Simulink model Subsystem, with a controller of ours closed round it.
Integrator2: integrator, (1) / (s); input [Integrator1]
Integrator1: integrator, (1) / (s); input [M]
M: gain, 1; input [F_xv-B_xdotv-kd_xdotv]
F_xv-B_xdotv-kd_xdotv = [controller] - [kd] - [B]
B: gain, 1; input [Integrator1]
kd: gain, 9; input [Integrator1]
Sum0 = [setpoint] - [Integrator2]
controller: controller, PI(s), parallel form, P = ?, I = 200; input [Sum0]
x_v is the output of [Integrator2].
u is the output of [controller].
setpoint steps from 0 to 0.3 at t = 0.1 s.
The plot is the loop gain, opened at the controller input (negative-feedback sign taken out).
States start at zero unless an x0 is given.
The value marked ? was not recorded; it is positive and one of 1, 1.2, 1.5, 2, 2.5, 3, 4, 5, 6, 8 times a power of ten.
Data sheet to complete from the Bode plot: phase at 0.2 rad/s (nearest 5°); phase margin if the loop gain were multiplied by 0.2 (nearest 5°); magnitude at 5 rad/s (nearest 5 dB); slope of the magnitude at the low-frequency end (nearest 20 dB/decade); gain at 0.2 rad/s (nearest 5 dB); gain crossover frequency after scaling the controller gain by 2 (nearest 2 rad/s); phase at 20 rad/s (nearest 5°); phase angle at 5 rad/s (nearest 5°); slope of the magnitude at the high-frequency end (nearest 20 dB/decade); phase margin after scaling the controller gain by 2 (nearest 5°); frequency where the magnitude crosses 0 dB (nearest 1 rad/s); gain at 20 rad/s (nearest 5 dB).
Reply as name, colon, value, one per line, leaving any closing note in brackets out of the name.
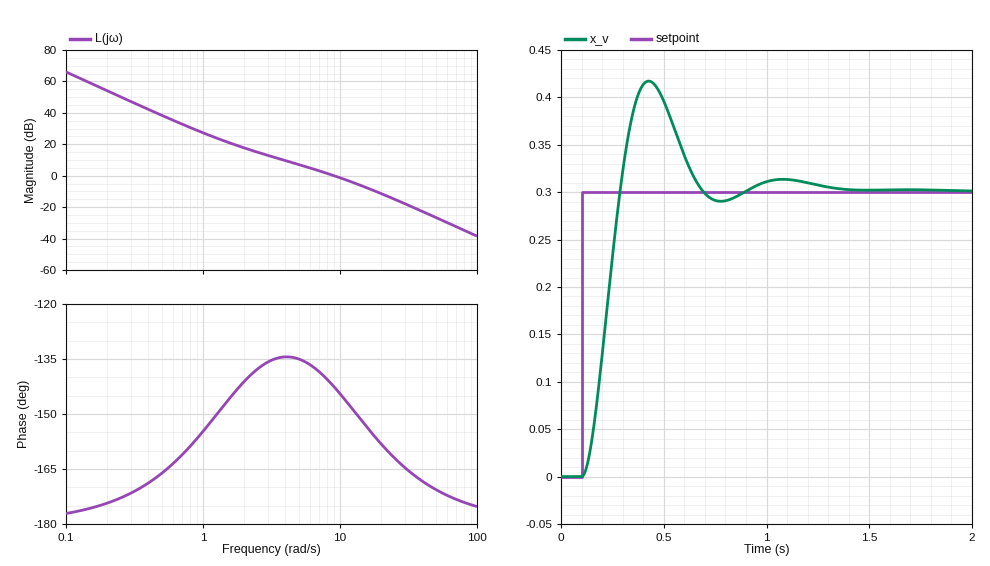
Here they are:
phase at 0.2 rad/s: -175°
phase margin if the loop gain were multiplied by 0.2: 45°
magnitude at 5 rad/s: 5 dB
slope of the magnitude at the low-frequency end: -40 dB/decade
gain at 0.2 rad/s: 55 dB
gain crossover frequency after scaling the controller gain by 2: 14 rad/s
phase at 20 rad/s: -160°
phase angle at 5 rad/s: -135°
slope of the magnitude at the high-frequency end: -40 dB/decade
phase margin after scaling the controller gain by 2: 30°
frequency where the magnitude crosses 0 dB: 9 rad/s
gain at 20 rad/s: -10 dB
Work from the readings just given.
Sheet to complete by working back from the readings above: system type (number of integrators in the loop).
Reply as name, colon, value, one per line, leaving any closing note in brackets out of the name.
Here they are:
system type: 2
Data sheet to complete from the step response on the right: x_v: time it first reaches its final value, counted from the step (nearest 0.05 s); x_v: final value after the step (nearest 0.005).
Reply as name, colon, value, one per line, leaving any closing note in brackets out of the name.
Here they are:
x_v: time it first reaches its final value, counted from the step: 0.20 s
x_v: final value after the step: 0.300
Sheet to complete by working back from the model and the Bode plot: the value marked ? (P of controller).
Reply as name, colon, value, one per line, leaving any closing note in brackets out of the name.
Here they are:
the value marked ?: 120
